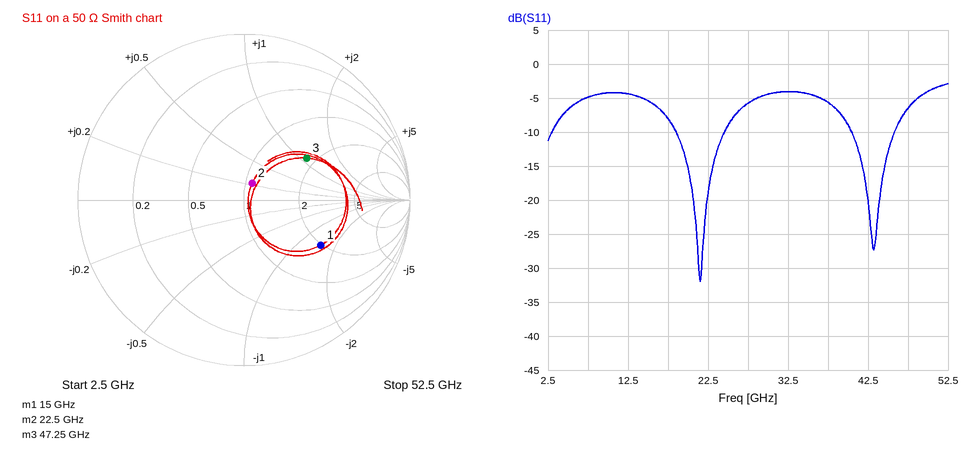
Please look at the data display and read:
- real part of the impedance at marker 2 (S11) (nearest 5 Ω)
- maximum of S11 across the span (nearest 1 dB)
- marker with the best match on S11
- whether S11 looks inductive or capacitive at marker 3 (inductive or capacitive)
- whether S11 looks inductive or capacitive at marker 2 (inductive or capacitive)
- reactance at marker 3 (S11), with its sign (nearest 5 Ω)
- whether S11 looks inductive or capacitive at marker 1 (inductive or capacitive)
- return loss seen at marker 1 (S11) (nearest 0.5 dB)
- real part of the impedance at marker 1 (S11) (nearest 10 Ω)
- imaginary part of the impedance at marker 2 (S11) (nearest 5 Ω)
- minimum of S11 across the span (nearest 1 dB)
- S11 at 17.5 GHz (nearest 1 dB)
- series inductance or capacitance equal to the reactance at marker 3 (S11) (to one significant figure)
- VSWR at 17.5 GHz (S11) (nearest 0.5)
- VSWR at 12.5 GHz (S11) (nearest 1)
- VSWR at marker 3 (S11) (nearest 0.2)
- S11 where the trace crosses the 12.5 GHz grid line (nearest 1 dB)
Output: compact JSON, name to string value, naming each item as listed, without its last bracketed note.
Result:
{"real part of the impedance at marker 2 (S11)": "55 Ω", "maximum of S11 across the span": "-3 dB", "marker with the best match on S11": "marker 2", "whether S11 looks inductive or capacitive at marker 3": "inductive", "whether S11 looks inductive or capacitive at marker 2": "inductive", "reactance at marker 3 (S11), with its sign": "+55 Ω", "whether S11 looks inductive or capacitive at marker 1": "capacitive", "return loss seen at marker 1 (S11)": "5.5 dB", "real part of the impedance at marker 1 (S11)": "100 Ω", "imaginary part of the impedance at marker 2 (S11)": "+10 Ω", "minimum of S11 across the span": "-32 dB", "S11 at 17.5 GHz": "-8 dB", "series inductance or capacitance equal to the reactance at marker 3 (S11)": "200 pH", "VSWR at 17.5 GHz (S11)": "2.5", "VSWR at 12.5 GHz (S11)": "4", "VSWR at marker 3 (S11)": "2.6", "S11 where the trace crosses the 12.5 GHz grid line": "-4 dB"}
